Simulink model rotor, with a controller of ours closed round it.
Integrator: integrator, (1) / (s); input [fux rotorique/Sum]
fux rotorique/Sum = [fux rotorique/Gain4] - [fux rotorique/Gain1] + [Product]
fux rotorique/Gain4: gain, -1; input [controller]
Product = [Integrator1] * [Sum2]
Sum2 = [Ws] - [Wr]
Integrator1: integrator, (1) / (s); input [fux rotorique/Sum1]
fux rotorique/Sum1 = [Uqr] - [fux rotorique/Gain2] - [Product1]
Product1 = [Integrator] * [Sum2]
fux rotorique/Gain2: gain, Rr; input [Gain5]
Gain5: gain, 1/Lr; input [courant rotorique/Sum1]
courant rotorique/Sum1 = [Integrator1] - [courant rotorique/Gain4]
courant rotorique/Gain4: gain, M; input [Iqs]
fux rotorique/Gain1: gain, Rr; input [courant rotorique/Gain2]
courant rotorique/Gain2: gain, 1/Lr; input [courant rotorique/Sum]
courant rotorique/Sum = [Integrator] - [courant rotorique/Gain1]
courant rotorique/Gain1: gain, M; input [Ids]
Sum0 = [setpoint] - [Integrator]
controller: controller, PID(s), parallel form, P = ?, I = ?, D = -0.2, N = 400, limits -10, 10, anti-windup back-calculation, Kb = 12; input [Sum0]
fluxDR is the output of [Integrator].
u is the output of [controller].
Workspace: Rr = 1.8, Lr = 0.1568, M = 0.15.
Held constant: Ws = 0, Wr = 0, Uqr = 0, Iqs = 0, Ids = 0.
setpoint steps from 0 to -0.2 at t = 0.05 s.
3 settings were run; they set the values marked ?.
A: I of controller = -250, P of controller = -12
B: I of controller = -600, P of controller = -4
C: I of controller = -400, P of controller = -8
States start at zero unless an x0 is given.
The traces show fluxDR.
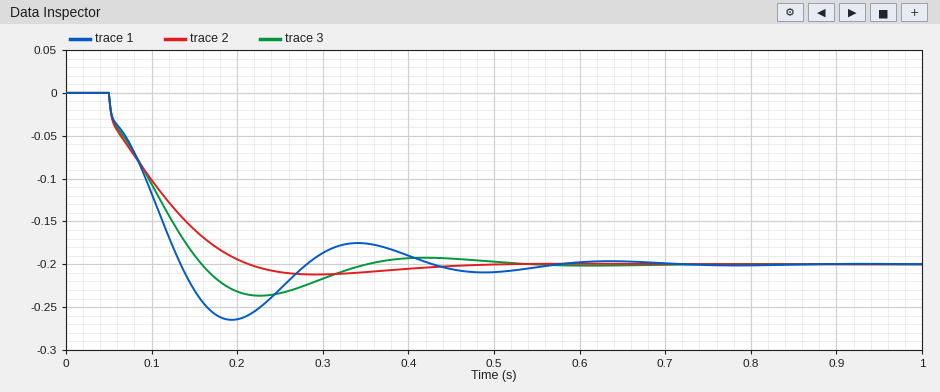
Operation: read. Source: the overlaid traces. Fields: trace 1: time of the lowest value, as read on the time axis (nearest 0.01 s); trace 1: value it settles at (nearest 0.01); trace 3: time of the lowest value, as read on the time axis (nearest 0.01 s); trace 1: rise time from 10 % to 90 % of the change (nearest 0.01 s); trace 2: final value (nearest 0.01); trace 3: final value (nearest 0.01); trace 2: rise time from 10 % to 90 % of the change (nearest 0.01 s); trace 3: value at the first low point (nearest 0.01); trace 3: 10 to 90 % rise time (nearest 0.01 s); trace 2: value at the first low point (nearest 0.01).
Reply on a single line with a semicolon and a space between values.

0.19 s; -0.20; 0.23 s; 0.07 s; -0.20; -0.20; 0.12 s; -0.24; 0.09 s; -0.21
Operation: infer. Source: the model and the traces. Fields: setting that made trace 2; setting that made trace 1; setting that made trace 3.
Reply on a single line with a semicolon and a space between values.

A; B; C
